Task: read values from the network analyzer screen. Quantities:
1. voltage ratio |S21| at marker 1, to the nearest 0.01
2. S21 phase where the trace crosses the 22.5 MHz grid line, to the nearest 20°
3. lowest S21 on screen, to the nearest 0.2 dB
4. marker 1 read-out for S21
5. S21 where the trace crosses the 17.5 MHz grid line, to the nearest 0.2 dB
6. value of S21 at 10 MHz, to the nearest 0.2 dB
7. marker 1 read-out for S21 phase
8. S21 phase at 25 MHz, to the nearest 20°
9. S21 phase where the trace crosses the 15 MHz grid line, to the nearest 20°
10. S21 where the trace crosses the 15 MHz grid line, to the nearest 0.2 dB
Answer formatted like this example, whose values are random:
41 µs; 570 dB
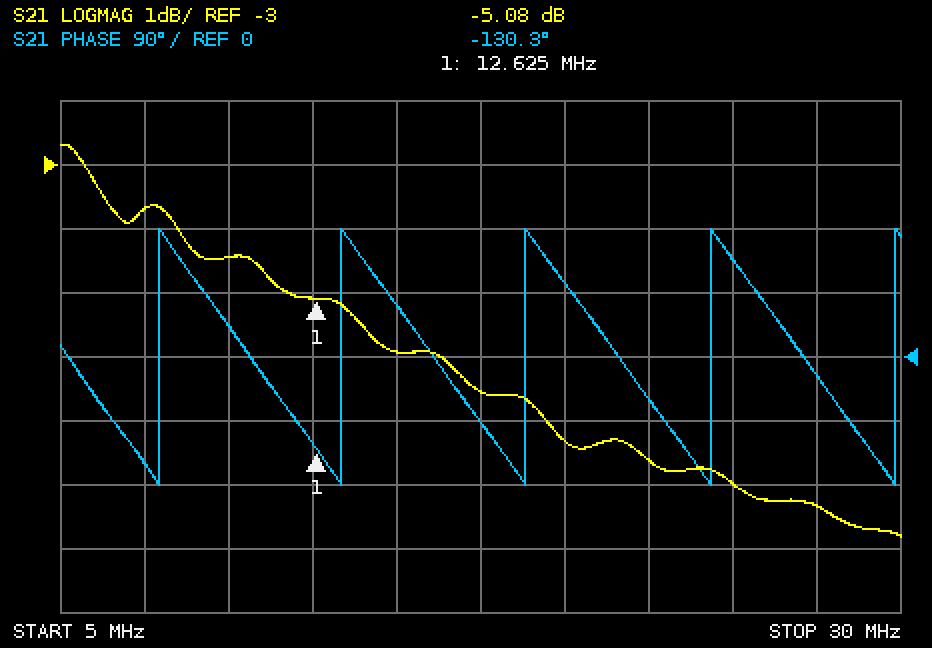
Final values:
0.56; -60°; -8.8 dB; -5.08 dB; -6.6 dB; -4.4 dB; -130.3°; 140°; 80°; -6.0 dB
